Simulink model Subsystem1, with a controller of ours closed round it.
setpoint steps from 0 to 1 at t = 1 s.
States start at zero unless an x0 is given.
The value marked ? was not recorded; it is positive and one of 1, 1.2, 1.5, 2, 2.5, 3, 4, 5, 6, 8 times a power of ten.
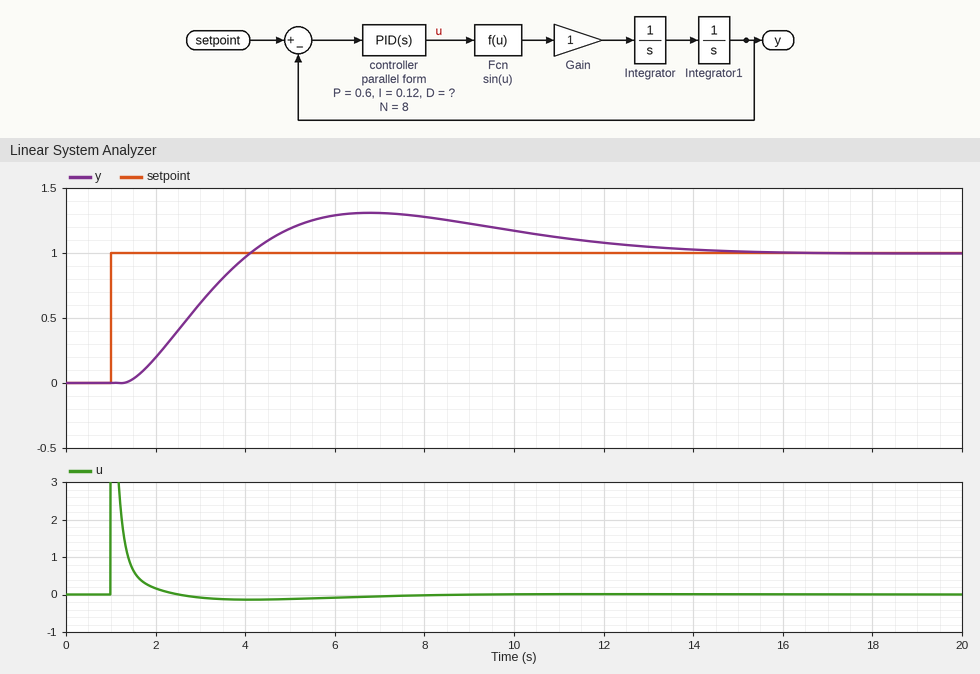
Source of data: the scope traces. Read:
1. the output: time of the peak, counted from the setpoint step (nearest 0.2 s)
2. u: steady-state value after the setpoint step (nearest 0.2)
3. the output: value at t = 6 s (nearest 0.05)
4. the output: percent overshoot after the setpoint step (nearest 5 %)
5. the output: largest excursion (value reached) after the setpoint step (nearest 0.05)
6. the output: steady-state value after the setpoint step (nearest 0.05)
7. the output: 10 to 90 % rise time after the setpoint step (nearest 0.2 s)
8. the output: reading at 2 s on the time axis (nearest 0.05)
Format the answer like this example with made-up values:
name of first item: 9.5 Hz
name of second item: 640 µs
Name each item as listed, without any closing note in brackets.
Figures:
the output: time of the peak, counted from the setpoint step: 5.8 s
u: steady-state value after the setpoint step: 0.0
the output: value at t = 6 s: 1.30
the output: percent overshoot after the setpoint step: 30 %
the output: largest excursion (value reached) after the setpoint step: 1.30
the output: steady-state value after the setpoint step: 1.00
the output: 10 to 90 % rise time after the setpoint step: 2.0 s
the output: reading at 2 s on the time axis: 0.20
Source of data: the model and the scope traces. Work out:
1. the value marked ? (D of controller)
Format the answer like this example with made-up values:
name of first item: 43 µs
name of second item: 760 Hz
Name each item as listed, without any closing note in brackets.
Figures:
the value marked ?: 1.2
